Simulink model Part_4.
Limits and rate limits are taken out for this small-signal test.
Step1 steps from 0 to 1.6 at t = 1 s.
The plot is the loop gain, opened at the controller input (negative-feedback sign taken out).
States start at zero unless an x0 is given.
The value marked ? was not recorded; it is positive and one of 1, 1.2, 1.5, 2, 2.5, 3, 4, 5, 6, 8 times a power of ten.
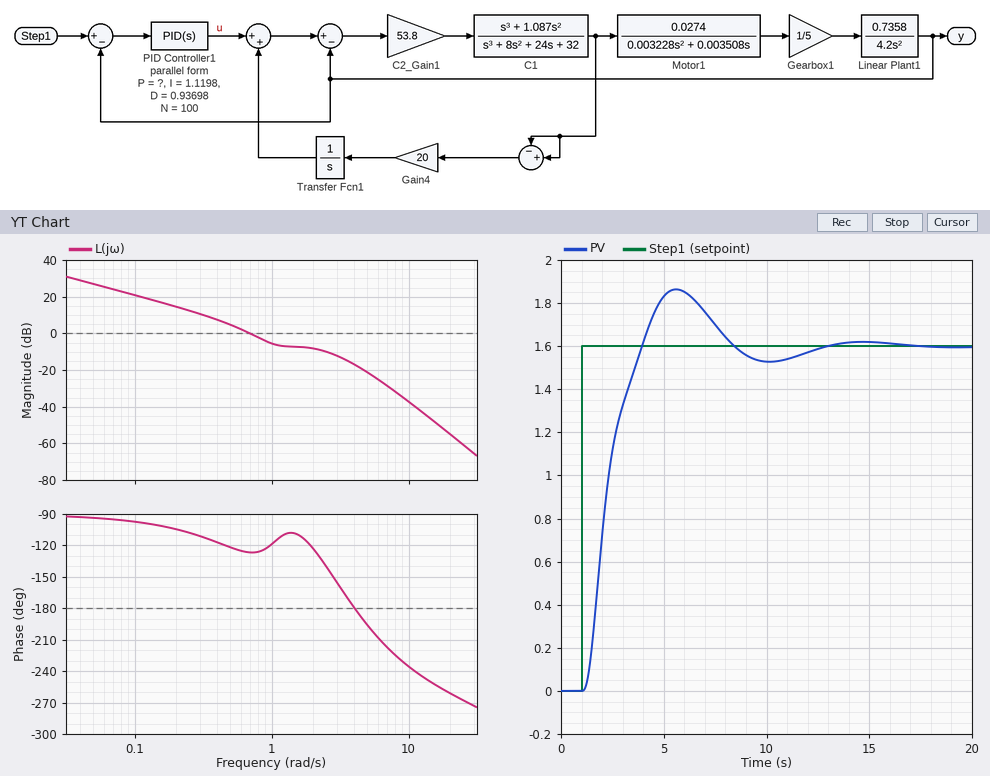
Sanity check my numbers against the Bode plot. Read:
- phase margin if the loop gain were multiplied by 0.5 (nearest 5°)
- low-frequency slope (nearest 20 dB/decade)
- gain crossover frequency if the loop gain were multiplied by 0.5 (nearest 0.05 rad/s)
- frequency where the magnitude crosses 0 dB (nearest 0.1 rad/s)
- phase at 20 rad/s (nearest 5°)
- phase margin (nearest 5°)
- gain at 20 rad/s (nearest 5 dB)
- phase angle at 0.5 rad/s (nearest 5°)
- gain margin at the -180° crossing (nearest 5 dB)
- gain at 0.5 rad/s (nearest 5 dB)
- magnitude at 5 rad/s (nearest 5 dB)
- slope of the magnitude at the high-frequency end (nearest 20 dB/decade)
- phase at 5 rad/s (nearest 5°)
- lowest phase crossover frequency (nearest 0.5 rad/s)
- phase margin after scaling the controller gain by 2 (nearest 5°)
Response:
60°
-20 dB/decade
0.45 rad/s
0.7 rad/s
-260°
55°
-55 dB
-120°
15 dB
5 dB
-20 dB
-60 dB/decade
-195°
4.0 rad/s
65°
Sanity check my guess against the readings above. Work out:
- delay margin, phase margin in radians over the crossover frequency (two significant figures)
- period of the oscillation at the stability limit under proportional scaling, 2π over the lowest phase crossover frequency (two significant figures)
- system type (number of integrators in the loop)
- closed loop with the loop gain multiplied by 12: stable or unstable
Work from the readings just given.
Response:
1.4 s
1.6 s
1
unstable
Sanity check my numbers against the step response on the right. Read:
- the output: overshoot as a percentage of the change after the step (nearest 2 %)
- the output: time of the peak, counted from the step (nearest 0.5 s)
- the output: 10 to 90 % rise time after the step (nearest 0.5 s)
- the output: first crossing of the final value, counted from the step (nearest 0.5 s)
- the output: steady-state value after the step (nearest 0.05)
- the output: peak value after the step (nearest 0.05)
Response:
16 %
4.5 s
2.0 s
3.0 s
1.60
1.85
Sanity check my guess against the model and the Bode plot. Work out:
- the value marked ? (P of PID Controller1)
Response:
0.8
